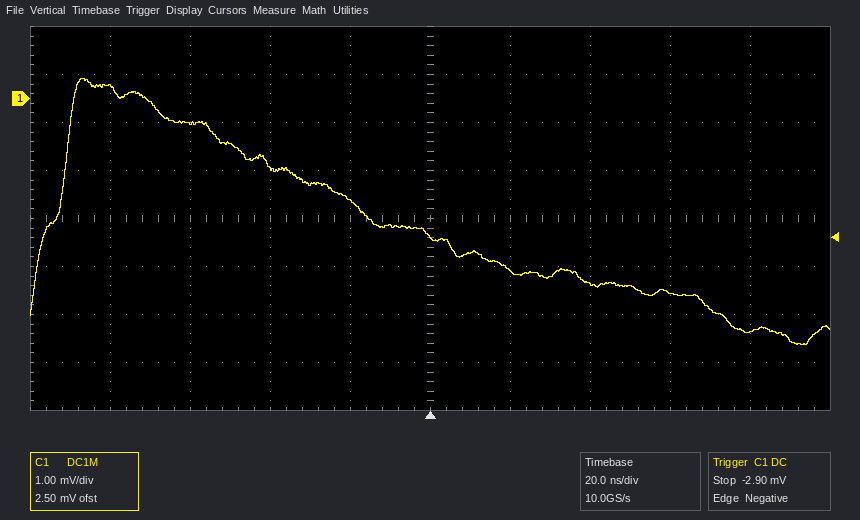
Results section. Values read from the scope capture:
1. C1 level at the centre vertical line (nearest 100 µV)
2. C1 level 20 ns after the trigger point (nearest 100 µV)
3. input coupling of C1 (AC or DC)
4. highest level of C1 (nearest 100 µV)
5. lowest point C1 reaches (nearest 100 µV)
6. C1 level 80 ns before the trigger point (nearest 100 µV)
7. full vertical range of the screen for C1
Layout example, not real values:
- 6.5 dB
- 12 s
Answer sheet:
- -2.9 mV
- -3.6 mV
- DC
- 400 µV
- -5.1 mV
- 200 µV
- 8 mV
